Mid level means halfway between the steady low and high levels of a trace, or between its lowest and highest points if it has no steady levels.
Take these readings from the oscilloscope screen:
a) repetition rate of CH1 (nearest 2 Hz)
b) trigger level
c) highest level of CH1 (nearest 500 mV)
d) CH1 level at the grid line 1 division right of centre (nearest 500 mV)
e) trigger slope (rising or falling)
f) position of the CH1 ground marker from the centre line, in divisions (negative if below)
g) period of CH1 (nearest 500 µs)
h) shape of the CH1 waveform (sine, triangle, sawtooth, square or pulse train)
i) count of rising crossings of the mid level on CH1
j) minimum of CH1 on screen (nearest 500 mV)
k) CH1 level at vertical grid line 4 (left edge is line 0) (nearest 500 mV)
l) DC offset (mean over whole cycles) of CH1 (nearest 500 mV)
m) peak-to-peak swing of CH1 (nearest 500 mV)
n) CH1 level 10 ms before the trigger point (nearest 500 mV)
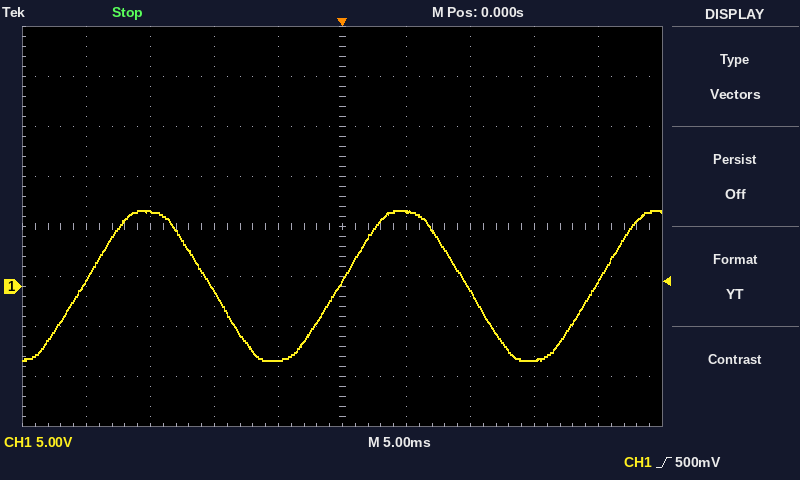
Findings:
50 Hz
500 mV
7.5 V
7.5 V
rising
-1.2 div
20.0 ms
sine
3
-7.5 V
-7.5 V
0.0 V
15.0 V
-500 mV
